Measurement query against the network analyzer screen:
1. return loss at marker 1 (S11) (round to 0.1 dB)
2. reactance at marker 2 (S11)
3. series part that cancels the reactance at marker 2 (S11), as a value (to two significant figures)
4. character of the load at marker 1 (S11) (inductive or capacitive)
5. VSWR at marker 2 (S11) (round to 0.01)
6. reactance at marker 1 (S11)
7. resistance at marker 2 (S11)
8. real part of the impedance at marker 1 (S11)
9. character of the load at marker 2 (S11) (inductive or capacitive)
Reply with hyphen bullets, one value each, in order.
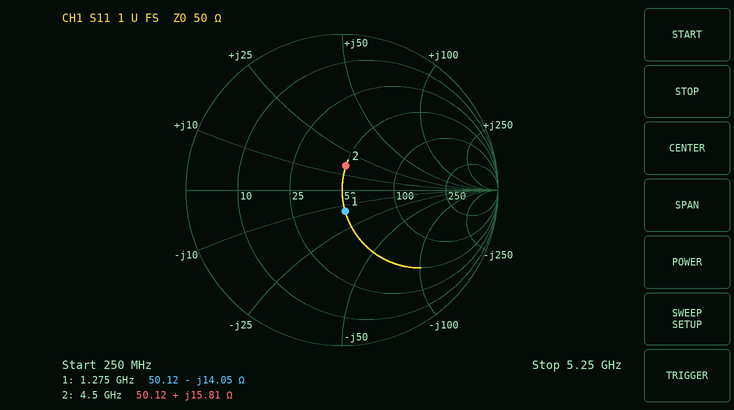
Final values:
- 17.1 dB
- +15.81 Ω
- 2.2 pF
- capacitive
- 1.37
- -14.05 Ω
- 50.12 Ω
- 50.12 Ω
- inductive
